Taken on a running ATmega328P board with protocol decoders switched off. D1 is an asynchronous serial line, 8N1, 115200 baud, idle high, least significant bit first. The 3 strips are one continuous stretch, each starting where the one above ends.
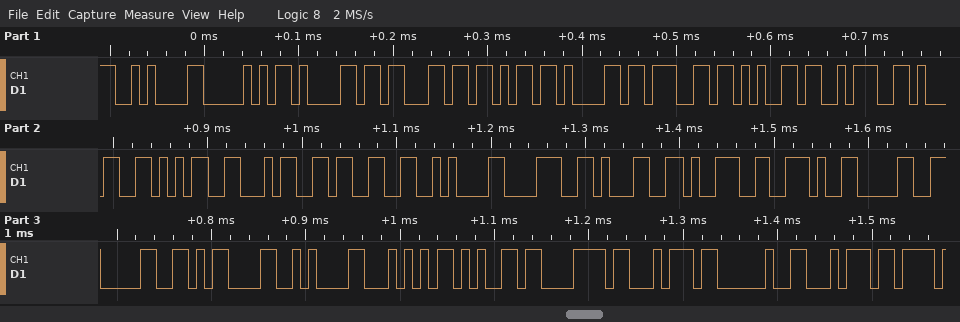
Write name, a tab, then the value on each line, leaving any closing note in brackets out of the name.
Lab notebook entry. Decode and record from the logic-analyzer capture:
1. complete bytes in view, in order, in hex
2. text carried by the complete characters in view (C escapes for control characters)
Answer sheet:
complete bytes in view, in order, in hex	0A 50 61 63 6B 61 67 65 3A 31 35 34 33 0A 38 31 39 2E 30 30 0D 0A 54 65 78 74 20 74
text carried by the complete characters in view	"\nPackage:1543\n819.00\r\nText t"
